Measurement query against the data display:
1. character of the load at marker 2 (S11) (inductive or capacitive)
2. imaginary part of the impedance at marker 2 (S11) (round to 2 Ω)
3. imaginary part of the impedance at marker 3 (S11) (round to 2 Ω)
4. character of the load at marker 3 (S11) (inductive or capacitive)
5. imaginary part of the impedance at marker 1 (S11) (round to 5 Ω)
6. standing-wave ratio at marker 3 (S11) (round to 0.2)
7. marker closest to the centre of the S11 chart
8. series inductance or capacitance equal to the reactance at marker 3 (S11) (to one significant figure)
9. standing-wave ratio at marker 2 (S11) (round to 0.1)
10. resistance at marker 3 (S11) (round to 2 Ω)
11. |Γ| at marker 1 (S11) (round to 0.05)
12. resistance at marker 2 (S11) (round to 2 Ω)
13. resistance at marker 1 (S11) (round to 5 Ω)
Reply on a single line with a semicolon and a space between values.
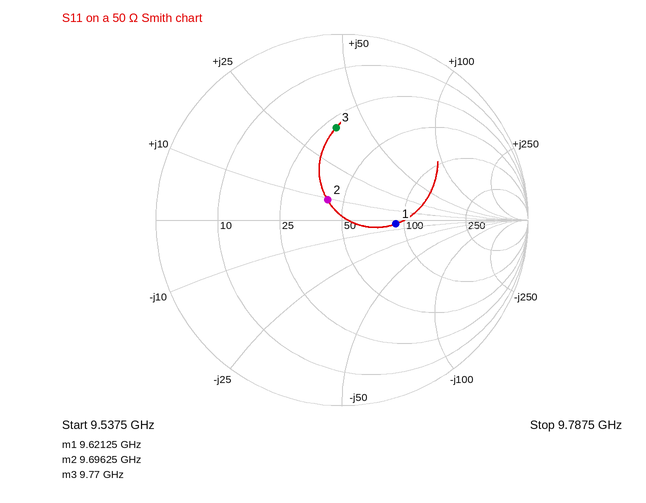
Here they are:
inductive; +10 Ω; +38 Ω; inductive; -5 Ω; 3.0; marker 2; 600 pH; 1.3; 28 Ω; 0.30; 42 Ω; 90 Ω
